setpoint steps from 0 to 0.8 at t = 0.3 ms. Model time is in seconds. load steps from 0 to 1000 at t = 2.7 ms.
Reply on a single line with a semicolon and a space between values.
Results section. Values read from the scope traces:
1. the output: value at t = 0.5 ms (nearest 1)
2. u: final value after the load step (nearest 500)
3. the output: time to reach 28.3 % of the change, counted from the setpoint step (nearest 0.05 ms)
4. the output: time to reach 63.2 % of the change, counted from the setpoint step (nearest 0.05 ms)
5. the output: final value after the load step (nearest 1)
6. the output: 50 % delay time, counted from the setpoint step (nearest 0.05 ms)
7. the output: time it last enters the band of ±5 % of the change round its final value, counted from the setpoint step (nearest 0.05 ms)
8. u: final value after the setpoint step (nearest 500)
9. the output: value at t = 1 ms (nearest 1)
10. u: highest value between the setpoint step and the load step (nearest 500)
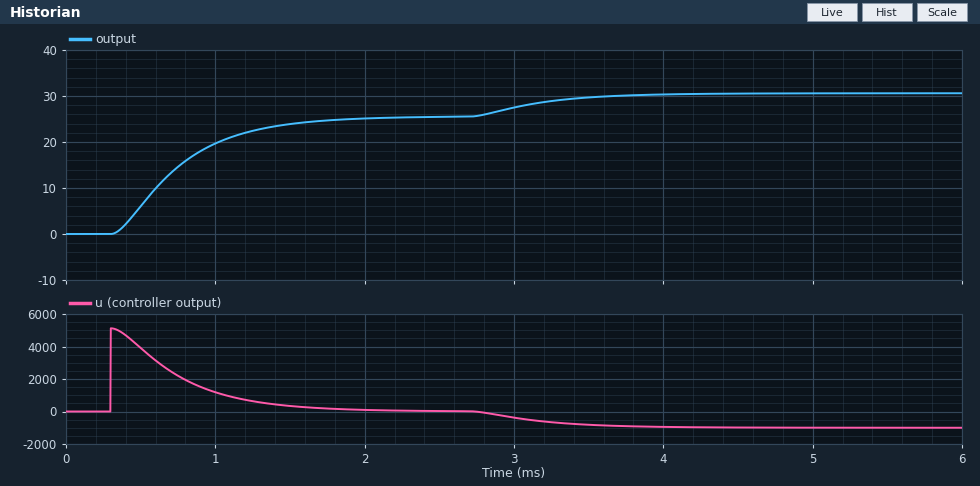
6; -1000; 0.25 ms; 0.50 ms; 31; 0.40 ms; 1.30 ms; 0; 20; 5000
